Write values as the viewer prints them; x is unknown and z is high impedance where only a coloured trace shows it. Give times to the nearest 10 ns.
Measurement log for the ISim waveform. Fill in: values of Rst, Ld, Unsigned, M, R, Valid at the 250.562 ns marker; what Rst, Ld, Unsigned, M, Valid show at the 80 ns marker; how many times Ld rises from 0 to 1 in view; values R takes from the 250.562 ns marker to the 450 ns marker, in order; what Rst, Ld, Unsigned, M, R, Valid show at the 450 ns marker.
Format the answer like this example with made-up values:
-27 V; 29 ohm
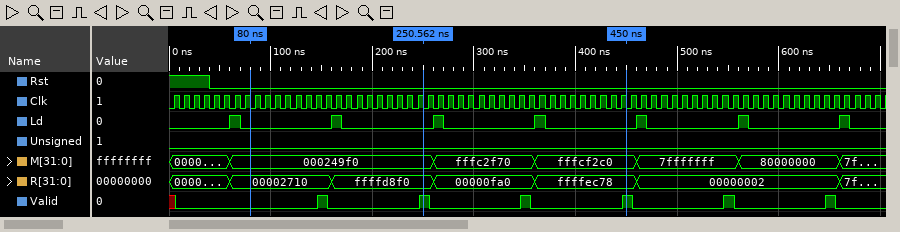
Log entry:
Rst=0, Ld=0, Unsigned=0, M=000249f0, R=ffffd8f0, Valid=1; Rst=0, Ld=0, Unsigned=0, M=000249f0, Valid=0; 7; ffffd8f0, 00000fa0, ffffec78; Rst=0, Ld=0, Unsigned=0, M=fffcf2c0, R=ffffec78, Valid=1
